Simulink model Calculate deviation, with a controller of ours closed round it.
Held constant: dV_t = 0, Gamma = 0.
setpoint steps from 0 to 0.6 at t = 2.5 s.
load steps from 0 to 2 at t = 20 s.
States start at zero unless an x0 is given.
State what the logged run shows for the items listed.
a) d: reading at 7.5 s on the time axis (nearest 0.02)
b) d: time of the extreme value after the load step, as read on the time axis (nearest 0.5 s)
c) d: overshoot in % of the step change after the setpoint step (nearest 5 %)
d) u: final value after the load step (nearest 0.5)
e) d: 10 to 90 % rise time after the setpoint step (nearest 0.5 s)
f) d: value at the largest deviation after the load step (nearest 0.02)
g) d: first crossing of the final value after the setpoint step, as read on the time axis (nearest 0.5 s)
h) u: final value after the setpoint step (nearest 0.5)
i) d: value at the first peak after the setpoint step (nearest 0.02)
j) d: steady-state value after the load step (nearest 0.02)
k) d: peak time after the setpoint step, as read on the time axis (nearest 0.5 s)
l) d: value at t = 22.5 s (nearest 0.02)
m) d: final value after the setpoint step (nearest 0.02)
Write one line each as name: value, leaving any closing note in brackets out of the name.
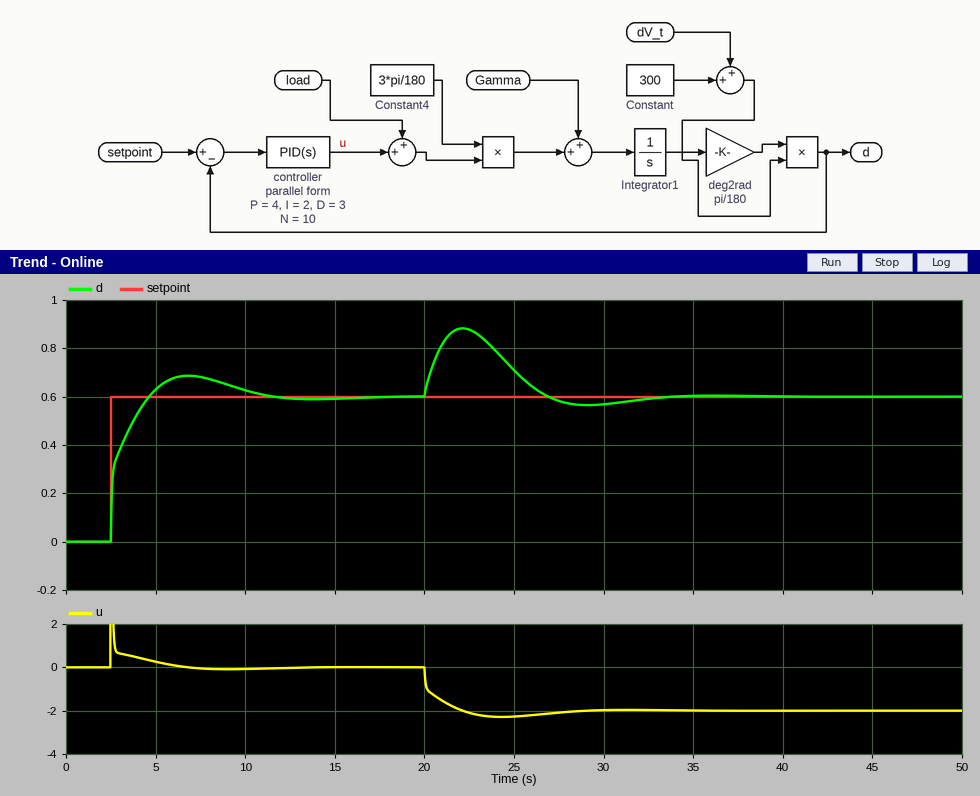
d: reading at 7.5 s on the time axis: 0.68
d: time of the extreme value after the load step, as read on the time axis: 22.0 s
d: overshoot in % of the step change after the setpoint step: 15 %
u: final value after the load step: -2.0
d: 10 to 90 % rise time after the setpoint step: 1.5 s
d: value at the largest deviation after the load step: 0.88
d: first crossing of the final value after the setpoint step, as read on the time axis: 4.5 s
u: final value after the setpoint step: 0.0
d: value at the first peak after the setpoint step: 0.68
d: steady-state value after the load step: 0.60
d: peak time after the setpoint step, as read on the time axis: 7.0 s
d: value at t = 22.5 s: 0.88
d: final value after the setpoint step: 0.60
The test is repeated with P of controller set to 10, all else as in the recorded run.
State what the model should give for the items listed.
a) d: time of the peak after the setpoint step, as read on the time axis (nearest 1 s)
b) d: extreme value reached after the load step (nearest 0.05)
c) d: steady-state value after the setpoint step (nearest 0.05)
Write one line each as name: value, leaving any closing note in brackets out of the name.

d: time of the peak after the setpoint step, as read on the time axis: 6 s
d: extreme value reached after the load step: 0.75
d: steady-state value after the setpoint step: 0.60
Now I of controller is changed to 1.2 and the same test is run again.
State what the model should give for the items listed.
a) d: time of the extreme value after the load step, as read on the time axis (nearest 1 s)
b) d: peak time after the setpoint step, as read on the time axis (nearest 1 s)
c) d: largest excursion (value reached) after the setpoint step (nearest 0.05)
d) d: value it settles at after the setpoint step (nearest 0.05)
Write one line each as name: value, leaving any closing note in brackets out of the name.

d: time of the extreme value after the load step, as read on the time axis: 23 s
d: peak time after the setpoint step, as read on the time axis: 8 s
d: largest excursion (value reached) after the setpoint step: 0.65
d: value it settles at after the setpoint step: 0.60
